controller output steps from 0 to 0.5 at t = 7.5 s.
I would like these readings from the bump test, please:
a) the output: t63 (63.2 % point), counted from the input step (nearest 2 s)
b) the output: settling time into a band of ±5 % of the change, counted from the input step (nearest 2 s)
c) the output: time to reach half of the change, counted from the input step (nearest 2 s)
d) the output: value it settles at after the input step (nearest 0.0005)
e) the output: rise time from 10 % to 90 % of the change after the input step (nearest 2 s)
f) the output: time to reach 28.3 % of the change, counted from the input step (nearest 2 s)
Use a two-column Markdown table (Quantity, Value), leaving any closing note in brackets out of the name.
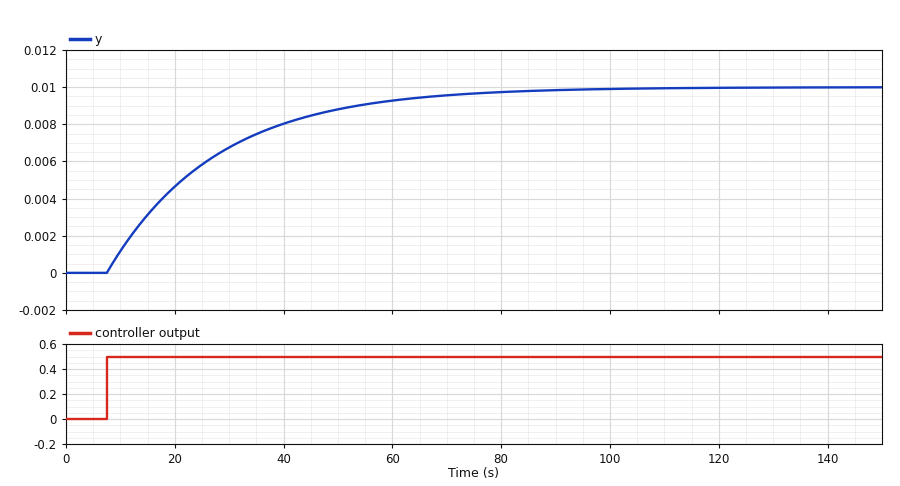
| Quantity | Value |
|---|---|
| the output: t63 (63.2 % point), counted from the input step | 20 s |
| the output: settling time into a band of ±5 % of the change, counted from the input step | 60 s |
| the output: time to reach half of the change, counted from the input step | 14 s |
| the output: value it settles at after the input step | 0.0100 |
| the output: rise time from 10 % to 90 % of the change after the input step | 44 s |
| the output: time to reach 28.3 % of the change, counted from the input step | 6 s |
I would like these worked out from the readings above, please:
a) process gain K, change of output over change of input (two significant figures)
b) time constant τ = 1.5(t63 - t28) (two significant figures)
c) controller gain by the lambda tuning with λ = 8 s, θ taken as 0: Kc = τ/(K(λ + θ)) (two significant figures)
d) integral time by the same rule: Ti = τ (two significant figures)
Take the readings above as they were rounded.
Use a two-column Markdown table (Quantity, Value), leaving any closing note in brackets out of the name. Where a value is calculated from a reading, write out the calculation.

| Quantity | Value |
|---|---|
| process gain K, change of output over change of input | (0.01 - 0) / 0.5 = 0.020 |
| time constant τ = 1.5(t63 - t28) | 1.5 × (20 - 6) = 21 s |
| controller gain by the lambda tuning with λ = 8 s, θ taken as 0: Kc = τ/(K(λ + θ)) | 21 / (0.02 × (8 + 0)) = 130 |
| integral time by the same rule: Ti = τ | 21 s |
